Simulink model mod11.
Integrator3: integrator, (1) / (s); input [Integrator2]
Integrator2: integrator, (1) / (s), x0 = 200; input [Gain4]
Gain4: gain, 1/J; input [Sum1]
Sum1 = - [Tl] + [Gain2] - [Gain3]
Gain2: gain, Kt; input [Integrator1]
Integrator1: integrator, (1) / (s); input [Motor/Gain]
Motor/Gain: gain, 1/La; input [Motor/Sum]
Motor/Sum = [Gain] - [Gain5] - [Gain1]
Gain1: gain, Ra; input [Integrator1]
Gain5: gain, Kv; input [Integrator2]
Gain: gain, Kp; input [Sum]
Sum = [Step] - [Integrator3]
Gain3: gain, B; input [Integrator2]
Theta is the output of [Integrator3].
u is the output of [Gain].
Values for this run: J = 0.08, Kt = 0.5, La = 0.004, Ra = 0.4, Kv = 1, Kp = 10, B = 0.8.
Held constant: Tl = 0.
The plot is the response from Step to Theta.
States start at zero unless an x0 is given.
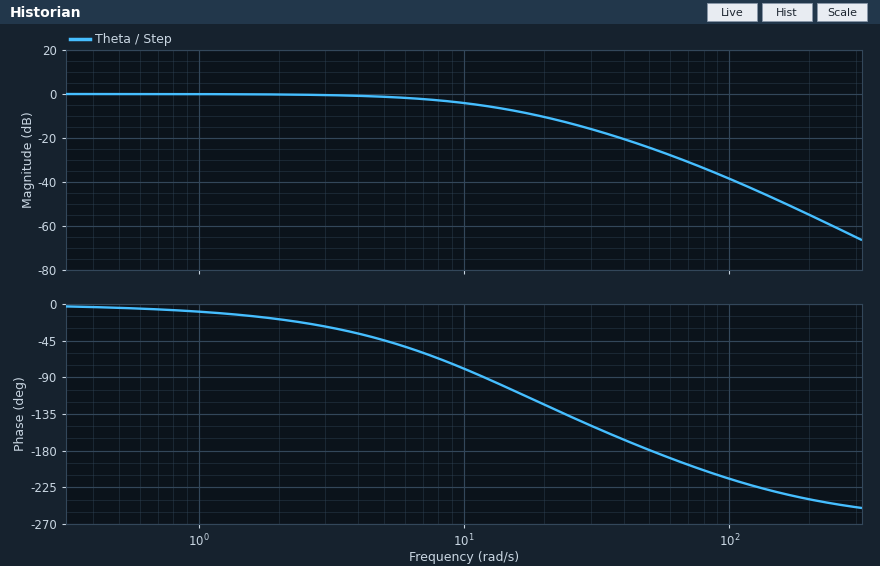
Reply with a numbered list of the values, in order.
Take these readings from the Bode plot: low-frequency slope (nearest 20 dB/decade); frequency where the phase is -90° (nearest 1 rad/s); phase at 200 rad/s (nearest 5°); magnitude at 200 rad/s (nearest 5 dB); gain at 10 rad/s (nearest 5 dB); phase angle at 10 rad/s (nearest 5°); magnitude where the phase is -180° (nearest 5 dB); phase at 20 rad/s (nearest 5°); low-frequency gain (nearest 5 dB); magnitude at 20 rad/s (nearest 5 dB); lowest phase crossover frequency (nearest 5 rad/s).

1. 0 dB/decade
2. 12 rad/s
3. -240°
4. -55 dB
5. -5 dB
6. -80°
7. -25 dB
8. -125°
9. 0 dB
10. -10 dB
11. 50 rad/s
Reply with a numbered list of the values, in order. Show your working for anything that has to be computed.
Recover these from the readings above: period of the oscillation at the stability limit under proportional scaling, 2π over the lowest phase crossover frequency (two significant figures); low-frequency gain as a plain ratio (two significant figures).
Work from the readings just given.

1. 2π / 50 = 0.13 s
2. 10^(0 / 20) = 1.0
